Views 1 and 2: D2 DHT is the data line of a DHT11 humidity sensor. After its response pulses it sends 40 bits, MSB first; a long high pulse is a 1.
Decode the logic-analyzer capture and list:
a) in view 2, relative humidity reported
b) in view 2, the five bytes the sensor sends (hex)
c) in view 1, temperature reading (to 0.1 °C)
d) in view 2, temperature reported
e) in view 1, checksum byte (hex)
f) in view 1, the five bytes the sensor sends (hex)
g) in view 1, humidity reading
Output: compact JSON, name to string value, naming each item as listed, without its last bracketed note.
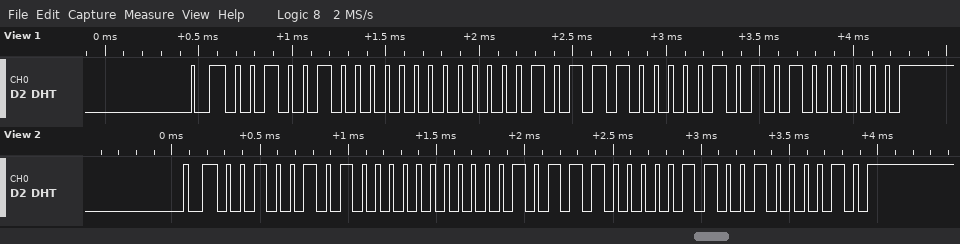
{"in view 2, relative humidity reported": "37 %", "in view 2, the five bytes the sensor sends": "25 00 17 06 42", "in view 1, temperature reading": "23.5 °C", "in view 2, temperature reported": "23.6 °C", "in view 1, checksum byte": "0x40", "in view 1, the five bytes the sensor sends": "24 00 17 05 40", "in view 1, humidity reading": "36 %"}
